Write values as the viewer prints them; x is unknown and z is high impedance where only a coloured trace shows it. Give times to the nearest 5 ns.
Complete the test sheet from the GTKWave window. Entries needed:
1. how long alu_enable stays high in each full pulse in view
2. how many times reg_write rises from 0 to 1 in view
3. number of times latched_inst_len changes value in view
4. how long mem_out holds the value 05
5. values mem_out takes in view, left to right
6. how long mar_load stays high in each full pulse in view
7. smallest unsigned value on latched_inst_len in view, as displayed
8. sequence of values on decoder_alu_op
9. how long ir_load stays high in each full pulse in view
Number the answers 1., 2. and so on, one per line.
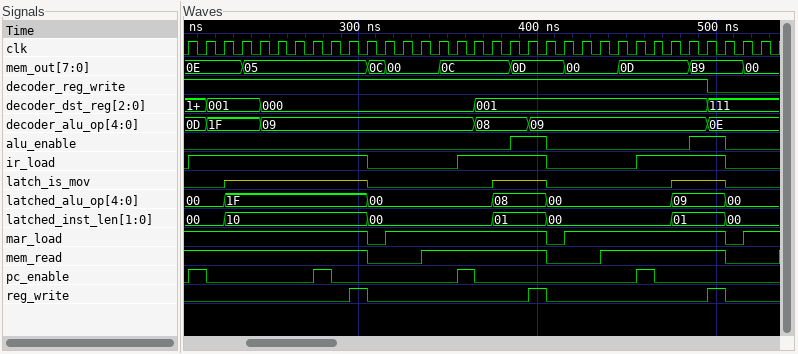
1. 20 ns, 20 ns
2. 3
3. 6
4. 70 ns
5. 0E, 05, 0C, 00, 0C, 0D, 00, 0D, B9, 00
6. 90 ns, 90 ns
7. 00
8. 0D, 1F, 09, 08, 09, 0E
9. 100 ns, 50 ns, 50 ns
